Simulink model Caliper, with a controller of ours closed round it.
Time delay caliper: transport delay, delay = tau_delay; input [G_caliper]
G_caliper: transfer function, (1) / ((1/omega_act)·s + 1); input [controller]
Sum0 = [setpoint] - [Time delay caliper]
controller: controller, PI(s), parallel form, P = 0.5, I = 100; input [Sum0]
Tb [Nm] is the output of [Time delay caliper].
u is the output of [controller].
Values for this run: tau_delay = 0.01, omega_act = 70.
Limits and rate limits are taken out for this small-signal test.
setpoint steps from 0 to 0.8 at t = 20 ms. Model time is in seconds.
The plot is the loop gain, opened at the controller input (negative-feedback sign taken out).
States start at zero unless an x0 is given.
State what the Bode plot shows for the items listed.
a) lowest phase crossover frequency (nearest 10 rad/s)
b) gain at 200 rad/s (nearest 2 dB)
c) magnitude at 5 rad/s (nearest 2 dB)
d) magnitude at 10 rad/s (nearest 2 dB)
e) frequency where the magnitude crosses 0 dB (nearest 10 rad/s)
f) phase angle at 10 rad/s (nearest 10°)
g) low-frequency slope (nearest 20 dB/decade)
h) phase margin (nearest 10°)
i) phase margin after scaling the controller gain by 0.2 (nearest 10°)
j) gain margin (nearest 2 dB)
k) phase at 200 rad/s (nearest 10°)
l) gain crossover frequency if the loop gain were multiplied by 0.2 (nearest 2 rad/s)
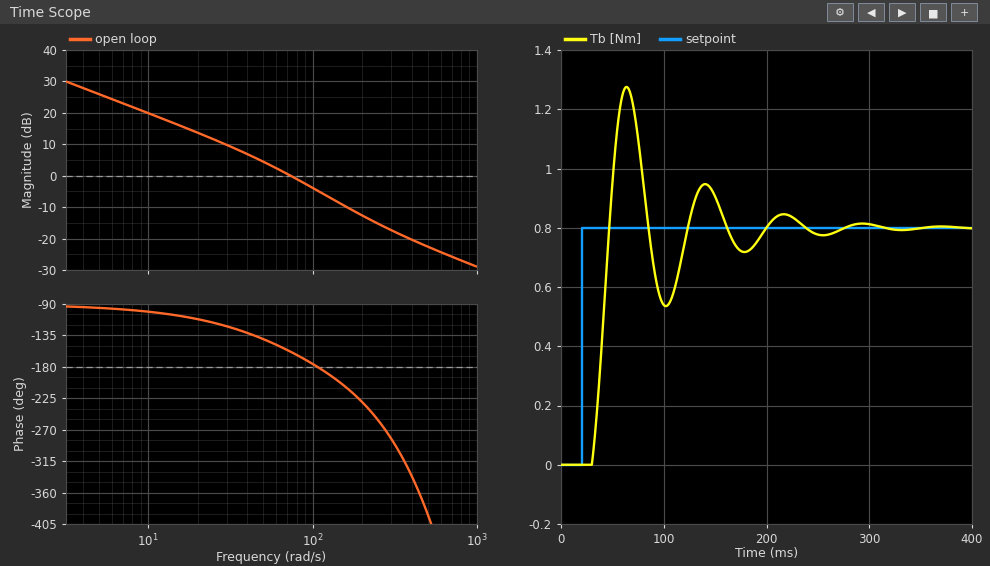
110 rad/s
-12 dB
26 dB
20 dB
70 rad/s
-100°
-20 dB/decade
20°
70°
4 dB
-230°
20 rad/s
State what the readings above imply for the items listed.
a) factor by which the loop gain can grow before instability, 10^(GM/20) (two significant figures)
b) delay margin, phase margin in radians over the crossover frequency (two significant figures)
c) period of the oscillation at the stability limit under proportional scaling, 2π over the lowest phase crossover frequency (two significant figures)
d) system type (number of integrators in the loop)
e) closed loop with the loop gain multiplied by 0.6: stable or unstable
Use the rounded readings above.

1.6
0.0050 s
0.057 s
1
stable
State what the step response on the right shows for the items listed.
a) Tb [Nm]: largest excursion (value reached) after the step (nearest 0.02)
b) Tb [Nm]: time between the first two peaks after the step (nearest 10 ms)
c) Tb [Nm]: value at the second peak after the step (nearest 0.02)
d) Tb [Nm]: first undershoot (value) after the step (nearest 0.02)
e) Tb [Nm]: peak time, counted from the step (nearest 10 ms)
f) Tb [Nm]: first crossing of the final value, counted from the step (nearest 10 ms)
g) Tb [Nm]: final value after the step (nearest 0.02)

1.28
80 ms
0.94
0.54
40 ms
30 ms
0.80
